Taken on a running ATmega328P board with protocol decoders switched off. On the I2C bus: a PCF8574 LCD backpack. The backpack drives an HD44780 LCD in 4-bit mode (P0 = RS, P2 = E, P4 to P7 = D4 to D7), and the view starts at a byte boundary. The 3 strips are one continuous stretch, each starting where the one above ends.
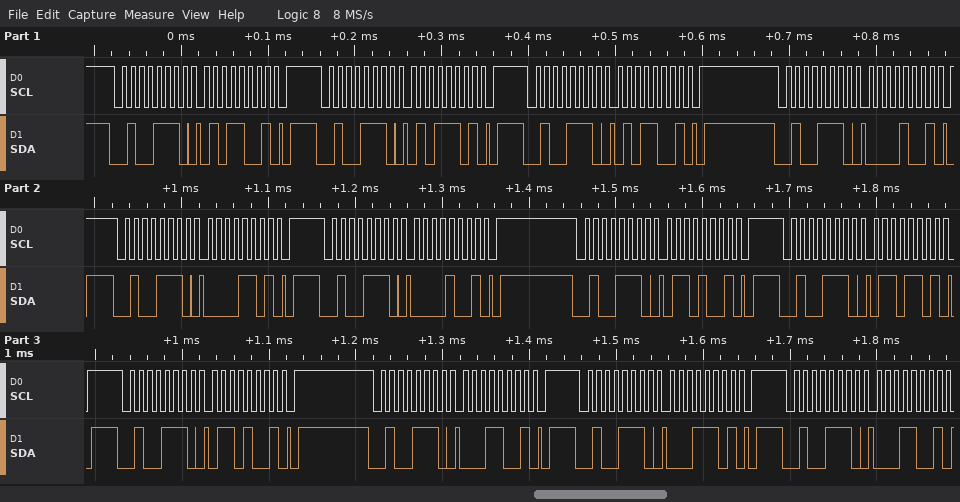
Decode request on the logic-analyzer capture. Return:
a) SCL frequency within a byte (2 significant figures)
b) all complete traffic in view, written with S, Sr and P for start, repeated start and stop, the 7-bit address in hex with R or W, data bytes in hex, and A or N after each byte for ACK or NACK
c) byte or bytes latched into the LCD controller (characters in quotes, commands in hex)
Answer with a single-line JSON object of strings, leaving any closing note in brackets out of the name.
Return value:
{"SCL frequency within a byte": "100 kHz", "all complete traffic in view, written with S, Sr and P for start, repeated start and stop, the 7-bit address in hex with R or W, data bytes in hex, and A or N after each byte for ACK or NACK": "S 27W A 59 A P S 27W A 5D A P S 27W A 59 A P S 27W A 09 A P S 27W A 0D A P S 27W A 09 A P S 27W A 69 A P S 27W A 6D A P S 27W A 69 A P S 27W A 19 A P S 27W A 1D A P S 27W A 19 A", "byte or bytes latched into the LCD controller": "'P' 'a'"}
